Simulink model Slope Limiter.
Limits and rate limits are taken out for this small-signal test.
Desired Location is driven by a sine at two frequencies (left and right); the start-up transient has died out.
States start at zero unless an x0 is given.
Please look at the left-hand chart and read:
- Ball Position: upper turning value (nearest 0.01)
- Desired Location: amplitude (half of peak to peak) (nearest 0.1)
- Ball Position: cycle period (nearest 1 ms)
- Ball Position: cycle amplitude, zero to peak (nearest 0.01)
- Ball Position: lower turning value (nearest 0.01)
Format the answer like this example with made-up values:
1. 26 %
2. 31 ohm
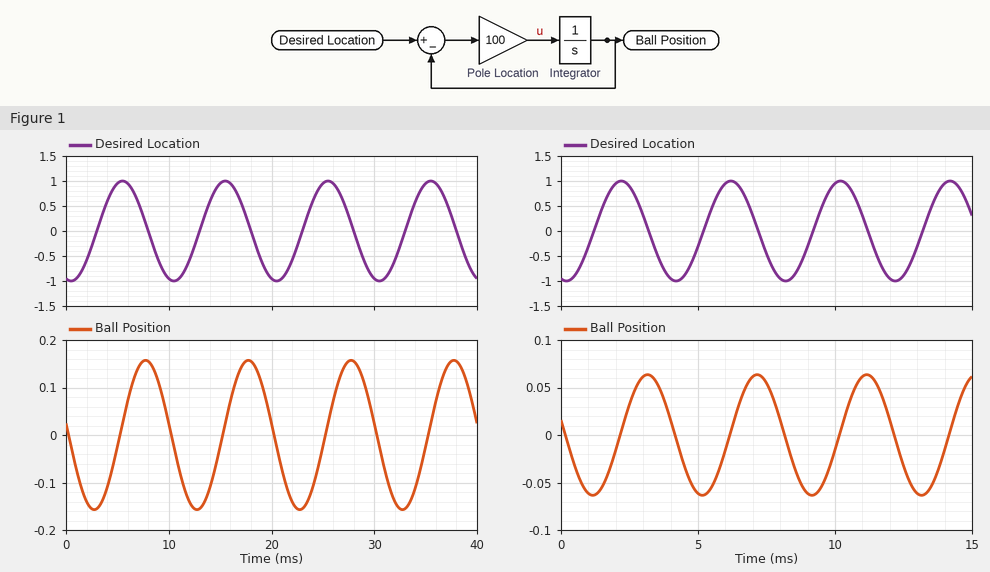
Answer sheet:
1. 0.16
2. 1.0
3. 10 ms
4. 0.16
5. -0.16
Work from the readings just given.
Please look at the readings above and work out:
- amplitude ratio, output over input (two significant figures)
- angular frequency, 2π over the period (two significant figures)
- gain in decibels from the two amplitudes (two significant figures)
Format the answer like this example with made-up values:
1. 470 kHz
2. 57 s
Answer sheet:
1. 0.16
2. 0.63 rad/ms
3. -16 dB
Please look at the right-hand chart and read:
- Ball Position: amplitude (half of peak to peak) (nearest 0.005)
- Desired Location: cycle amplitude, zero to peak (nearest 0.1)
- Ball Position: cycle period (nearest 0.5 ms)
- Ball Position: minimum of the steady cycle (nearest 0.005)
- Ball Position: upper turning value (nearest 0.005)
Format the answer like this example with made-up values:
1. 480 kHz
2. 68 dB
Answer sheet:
1. 0.065
2. 1.0
3. 4.0 ms
4. -0.065
5. 0.065
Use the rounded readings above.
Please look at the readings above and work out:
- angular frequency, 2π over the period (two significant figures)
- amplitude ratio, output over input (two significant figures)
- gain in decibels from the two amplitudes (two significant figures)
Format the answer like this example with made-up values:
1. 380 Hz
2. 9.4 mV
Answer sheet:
1. 1.6 rad/ms
2. 0.065
3. -24 dB
